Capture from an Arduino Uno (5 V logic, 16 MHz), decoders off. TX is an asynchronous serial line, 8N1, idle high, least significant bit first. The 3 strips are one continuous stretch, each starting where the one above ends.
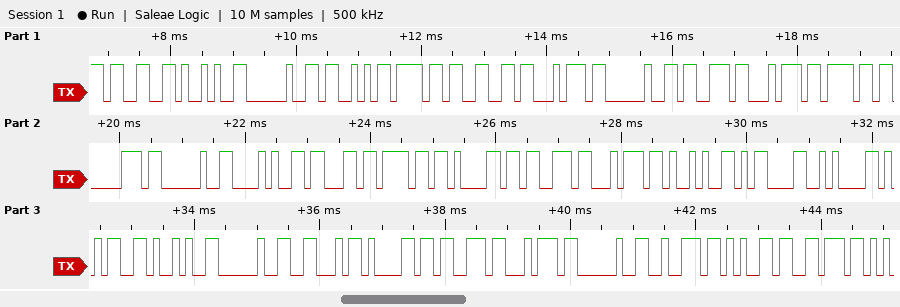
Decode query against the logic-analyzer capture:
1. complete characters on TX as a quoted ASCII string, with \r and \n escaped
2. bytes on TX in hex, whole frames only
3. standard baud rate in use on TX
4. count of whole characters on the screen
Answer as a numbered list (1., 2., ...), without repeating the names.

1. "3) Soft stop (coast)\r\n5) Fast rev"
2. 33 29 20 53 6F 66 74 20 73 74 6F 70 20 28 63 6F 61 73 74 29 0D 0A 35 29 20 46 61 73 74 20 72 65 76
3. 9600 baud
4. 33
